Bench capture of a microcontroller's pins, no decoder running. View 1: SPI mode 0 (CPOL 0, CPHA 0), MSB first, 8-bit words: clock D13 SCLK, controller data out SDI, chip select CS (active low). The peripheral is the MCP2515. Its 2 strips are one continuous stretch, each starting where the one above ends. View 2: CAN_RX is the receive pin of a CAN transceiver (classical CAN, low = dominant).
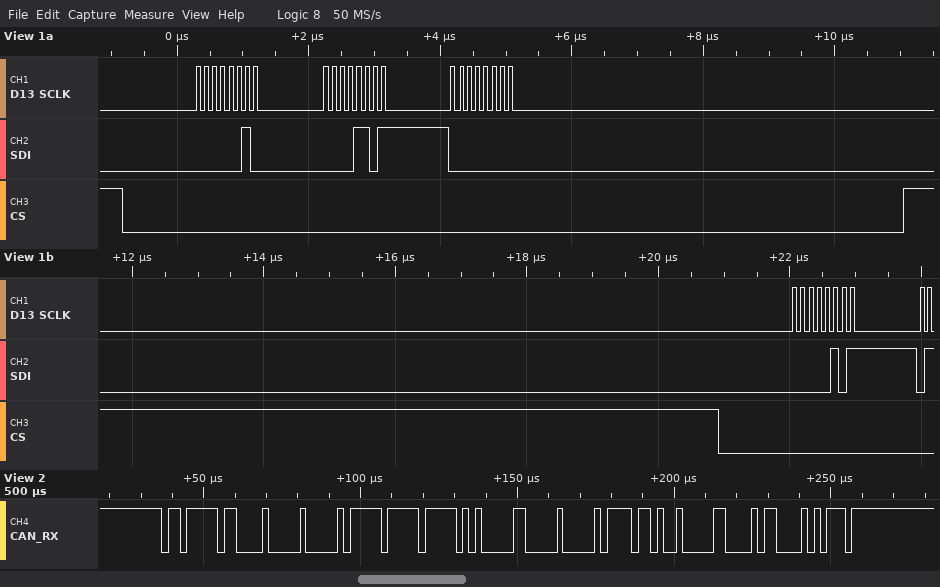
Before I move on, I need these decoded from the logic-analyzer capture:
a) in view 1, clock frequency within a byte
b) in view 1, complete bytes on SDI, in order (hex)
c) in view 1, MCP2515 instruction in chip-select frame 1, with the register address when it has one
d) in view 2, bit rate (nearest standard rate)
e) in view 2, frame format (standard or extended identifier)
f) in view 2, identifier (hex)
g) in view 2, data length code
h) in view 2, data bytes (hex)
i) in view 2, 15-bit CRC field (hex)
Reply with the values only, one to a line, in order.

8 MHz
02 0D 00 05
WRITE 0x0D
500 kbit/s
standard
0x6FE
8
00 FF FF 41 00 1E D2 08
0x2C2B
